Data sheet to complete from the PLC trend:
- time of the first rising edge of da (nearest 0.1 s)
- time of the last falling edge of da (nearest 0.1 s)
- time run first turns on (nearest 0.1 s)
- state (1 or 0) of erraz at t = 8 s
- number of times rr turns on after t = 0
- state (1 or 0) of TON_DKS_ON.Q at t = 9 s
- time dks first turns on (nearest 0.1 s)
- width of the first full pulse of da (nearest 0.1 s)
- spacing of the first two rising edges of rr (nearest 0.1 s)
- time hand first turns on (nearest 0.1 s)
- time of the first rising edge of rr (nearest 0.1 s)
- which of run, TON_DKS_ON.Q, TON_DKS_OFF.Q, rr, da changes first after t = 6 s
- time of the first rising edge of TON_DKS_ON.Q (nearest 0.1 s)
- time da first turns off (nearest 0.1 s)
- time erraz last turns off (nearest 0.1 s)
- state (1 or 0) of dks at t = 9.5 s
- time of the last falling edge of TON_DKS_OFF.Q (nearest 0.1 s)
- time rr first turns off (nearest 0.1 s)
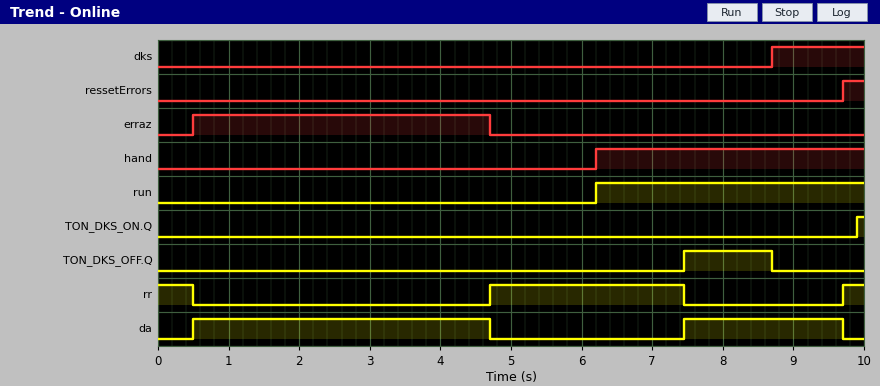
0.5 s
9.7 s
6.2 s
0
2
0
8.7 s
4.2 s
5.0 s
6.2 s
4.7 s
run
9.9 s
4.7 s
4.7 s
1
8.7 s
0.5 s
